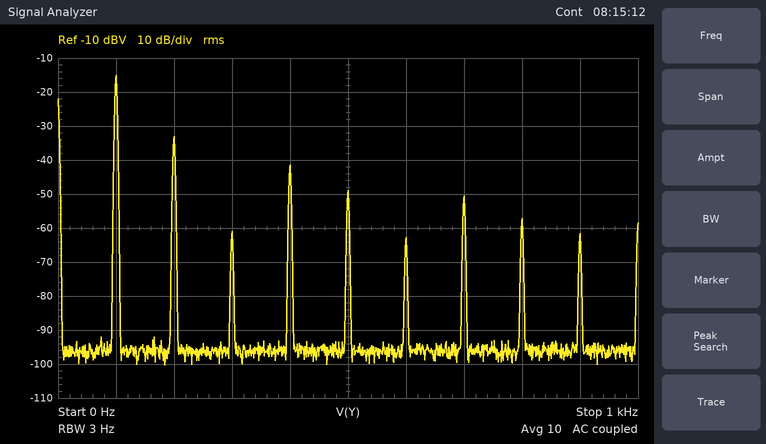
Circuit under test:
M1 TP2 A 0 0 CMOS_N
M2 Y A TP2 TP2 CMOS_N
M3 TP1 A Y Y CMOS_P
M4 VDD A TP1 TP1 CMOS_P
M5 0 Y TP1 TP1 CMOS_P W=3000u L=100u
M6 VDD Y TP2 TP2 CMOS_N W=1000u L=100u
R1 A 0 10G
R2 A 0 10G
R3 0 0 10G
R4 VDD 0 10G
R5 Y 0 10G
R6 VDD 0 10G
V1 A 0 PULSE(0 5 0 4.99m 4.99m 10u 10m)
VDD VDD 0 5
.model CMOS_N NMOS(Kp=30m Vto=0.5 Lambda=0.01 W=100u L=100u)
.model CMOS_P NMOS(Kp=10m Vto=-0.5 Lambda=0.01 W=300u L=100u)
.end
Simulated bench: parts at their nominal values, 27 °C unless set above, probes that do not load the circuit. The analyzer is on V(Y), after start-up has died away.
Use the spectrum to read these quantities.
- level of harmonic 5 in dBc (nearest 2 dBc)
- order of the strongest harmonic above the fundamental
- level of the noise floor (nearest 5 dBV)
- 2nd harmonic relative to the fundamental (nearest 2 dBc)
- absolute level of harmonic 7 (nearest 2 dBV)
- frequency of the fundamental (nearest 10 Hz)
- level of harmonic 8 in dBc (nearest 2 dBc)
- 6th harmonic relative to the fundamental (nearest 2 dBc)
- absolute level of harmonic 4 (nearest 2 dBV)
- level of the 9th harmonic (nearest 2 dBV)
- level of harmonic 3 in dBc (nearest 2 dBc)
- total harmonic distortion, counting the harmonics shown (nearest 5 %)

-34 dBc
2
-95 dBV
-18 dBc
-50 dBV
100 Hz
-42 dBc
-48 dBc
-42 dBV
-62 dBV
-46 dBc
15 %
